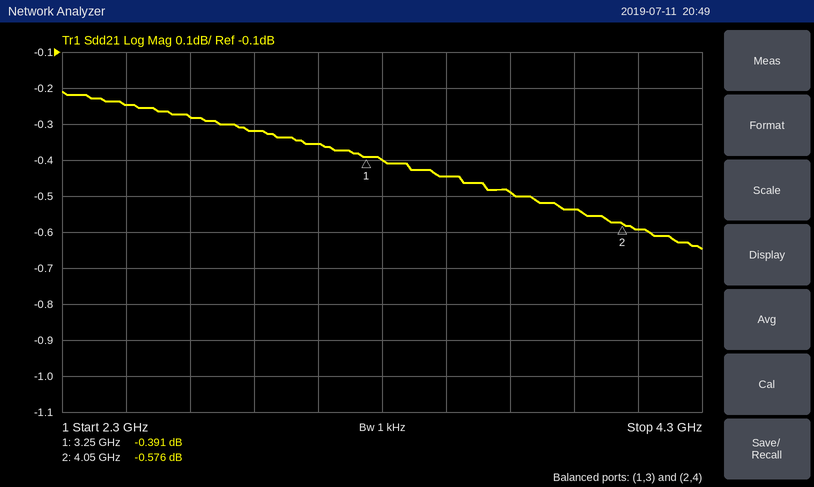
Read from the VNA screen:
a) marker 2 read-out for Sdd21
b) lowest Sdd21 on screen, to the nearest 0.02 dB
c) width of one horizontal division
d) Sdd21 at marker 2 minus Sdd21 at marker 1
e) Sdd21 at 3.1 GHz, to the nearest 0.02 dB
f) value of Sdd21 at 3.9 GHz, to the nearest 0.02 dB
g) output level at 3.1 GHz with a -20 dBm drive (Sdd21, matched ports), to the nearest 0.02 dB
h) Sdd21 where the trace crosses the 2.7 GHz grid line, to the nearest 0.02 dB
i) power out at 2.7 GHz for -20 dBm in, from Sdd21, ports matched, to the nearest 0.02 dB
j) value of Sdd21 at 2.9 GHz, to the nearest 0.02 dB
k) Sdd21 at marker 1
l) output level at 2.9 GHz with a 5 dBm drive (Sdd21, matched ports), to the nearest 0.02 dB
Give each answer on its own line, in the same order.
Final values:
-0.576 dB
-0.64 dB
200 MHz
-0.185 dB
-0.36 dB
-0.54 dB
-20.36 dBm
-0.28 dB
-20.28 dBm
-0.32 dB
-0.391 dB
4.68 dBm
